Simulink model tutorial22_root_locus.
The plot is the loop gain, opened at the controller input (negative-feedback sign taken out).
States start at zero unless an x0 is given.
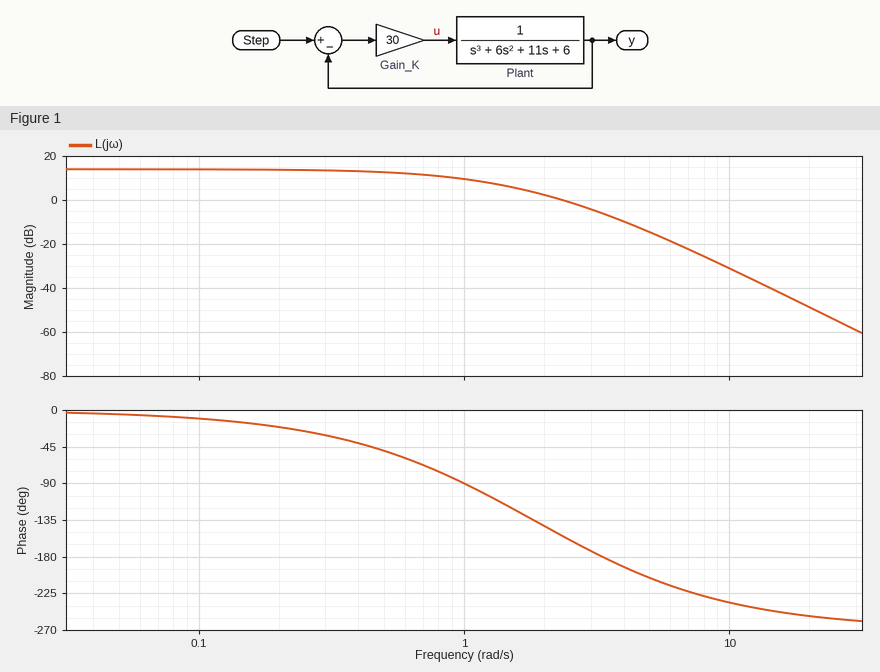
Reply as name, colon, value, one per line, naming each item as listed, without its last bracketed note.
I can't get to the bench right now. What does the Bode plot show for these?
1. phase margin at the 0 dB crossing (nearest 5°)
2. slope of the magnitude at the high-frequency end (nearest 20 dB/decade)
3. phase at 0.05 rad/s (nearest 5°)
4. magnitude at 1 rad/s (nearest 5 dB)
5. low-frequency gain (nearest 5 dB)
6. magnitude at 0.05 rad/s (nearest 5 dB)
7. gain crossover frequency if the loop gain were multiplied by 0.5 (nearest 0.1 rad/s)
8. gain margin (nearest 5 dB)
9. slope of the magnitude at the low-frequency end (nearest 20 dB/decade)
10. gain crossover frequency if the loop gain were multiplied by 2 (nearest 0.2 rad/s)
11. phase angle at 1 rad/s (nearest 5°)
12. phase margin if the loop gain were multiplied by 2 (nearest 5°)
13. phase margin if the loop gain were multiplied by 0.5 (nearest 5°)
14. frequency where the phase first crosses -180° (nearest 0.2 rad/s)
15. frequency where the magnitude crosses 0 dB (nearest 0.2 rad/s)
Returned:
phase margin at the 0 dB crossing: 25°
slope of the magnitude at the high-frequency end: -60 dB/decade
phase at 0.05 rad/s: -5°
magnitude at 1 rad/s: 10 dB
low-frequency gain: 15 dB
magnitude at 0.05 rad/s: 15 dB
gain crossover frequency if the loop gain were multiplied by 0.5: 1.5 rad/s
gain margin: 5 dB
slope of the magnitude at the low-frequency end: 0 dB/decade
gain crossover frequency if the loop gain were multiplied by 2: 3.4 rad/s
phase angle at 1 rad/s: -90°
phase margin if the loop gain were multiplied by 2: 0°
phase margin if the loop gain were multiplied by 0.5: 60°
frequency where the phase first crosses -180°: 3.4 rad/s
frequency where the magnitude crosses 0 dB: 2.4 rad/s
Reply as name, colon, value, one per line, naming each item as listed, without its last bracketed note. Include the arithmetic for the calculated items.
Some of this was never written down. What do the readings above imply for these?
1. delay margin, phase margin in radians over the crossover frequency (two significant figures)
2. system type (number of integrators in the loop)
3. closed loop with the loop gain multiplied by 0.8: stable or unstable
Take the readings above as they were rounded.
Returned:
delay margin, phase margin in radians over the crossover frequency: 25 × π / 180 / 2.4 = 0.18 s
system type: 0
closed loop with the loop gain multiplied by 0.8: stable or unstable: stable
